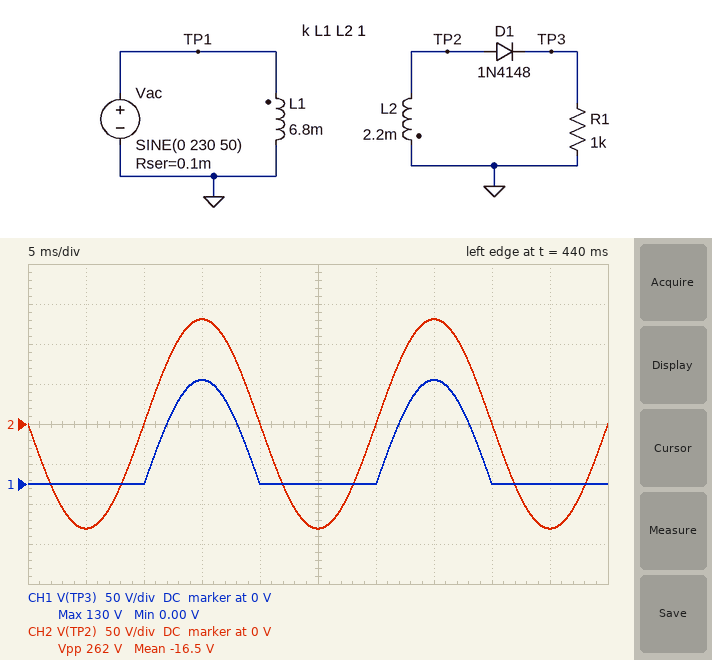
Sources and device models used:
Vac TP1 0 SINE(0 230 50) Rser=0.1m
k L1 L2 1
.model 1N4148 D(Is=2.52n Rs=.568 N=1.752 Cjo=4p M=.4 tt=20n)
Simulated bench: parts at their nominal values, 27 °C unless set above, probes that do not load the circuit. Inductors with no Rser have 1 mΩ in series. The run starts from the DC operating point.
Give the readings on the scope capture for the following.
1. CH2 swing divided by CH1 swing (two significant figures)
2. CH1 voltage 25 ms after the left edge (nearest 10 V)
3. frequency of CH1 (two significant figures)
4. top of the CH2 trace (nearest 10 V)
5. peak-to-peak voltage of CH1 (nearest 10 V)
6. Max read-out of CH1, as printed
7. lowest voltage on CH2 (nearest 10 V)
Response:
2.0
0 V
50 Hz
130 V
130 V
130 V
-130 V
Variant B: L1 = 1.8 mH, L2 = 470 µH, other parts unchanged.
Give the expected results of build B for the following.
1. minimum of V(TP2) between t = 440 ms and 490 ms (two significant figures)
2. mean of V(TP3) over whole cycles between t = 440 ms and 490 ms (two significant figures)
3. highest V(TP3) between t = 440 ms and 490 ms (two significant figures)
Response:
-120 V
37 V
120 V
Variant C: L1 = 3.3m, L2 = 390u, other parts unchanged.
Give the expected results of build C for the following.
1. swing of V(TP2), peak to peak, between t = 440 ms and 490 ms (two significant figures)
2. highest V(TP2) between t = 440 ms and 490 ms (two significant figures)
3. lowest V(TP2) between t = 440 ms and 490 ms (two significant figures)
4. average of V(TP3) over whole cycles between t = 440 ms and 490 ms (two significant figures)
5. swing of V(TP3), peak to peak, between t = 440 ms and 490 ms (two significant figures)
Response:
160 V
79 V
-79 V
25 V
78 V
